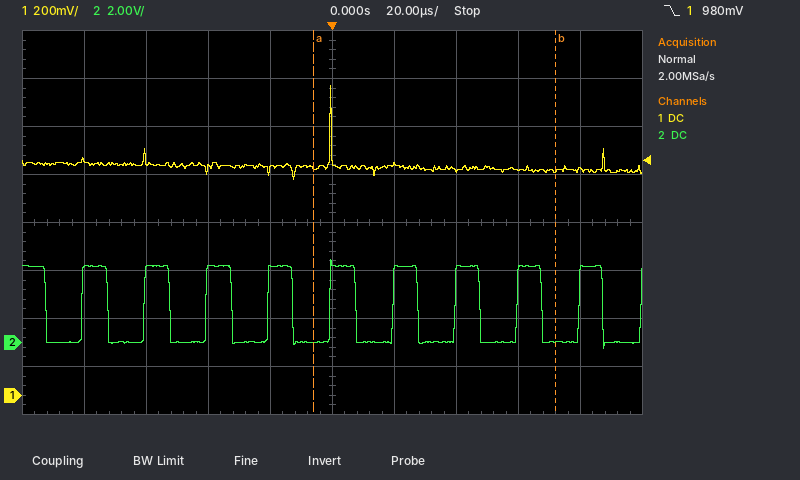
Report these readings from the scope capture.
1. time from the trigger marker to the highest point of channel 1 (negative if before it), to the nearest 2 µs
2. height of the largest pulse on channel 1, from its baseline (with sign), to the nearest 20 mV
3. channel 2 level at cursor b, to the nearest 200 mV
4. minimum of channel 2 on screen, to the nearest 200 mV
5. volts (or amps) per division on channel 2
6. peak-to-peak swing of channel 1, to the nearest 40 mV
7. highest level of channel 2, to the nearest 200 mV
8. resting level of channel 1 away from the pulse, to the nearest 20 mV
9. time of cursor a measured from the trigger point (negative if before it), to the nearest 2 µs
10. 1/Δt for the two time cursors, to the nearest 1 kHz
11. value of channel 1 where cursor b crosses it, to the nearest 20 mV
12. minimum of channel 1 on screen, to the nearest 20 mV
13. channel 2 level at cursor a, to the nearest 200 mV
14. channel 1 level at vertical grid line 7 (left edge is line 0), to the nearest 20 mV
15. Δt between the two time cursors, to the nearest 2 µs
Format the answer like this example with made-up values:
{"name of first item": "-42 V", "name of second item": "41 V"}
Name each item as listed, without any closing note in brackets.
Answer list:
{"time from the trigger marker to the highest point of channel 1 (negative if before it), to the nearest 2 µs": "0 µs", "height of the largest pulse on channel 1, from its baseline (with sign), to the nearest 20 mV": "+340 mV", "channel 2 level at cursor b, to the nearest 200 mV": "0.0 V", "minimum of channel 2 on screen, to the nearest 200 mV": "-200 mV", "volts (or amps) per division on channel 2": "2 V", "peak-to-peak swing of channel 1, to the nearest 40 mV": "400 mV", "highest level of channel 2, to the nearest 200 mV": "3.4 V", "resting level of channel 1 away from the pulse, to the nearest 20 mV": "960 mV", "time of cursor a measured from the trigger point (negative if before it), to the nearest 2 µs": "-6 µs", "1/Δt for the two time cursors, to the nearest 1 kHz": "13 kHz", "value of channel 1 where cursor b crosses it, to the nearest 20 mV": "940 mV", "minimum of channel 1 on screen, to the nearest 20 mV": "900 mV", "channel 2 level at cursor a, to the nearest 200 mV": "0.0 V", "channel 1 level at vertical grid line 7 (left edge is line 0), to the nearest 20 mV": "940 mV", "Δt between the two time cursors, to the nearest 2 µs": "78 µs"}
